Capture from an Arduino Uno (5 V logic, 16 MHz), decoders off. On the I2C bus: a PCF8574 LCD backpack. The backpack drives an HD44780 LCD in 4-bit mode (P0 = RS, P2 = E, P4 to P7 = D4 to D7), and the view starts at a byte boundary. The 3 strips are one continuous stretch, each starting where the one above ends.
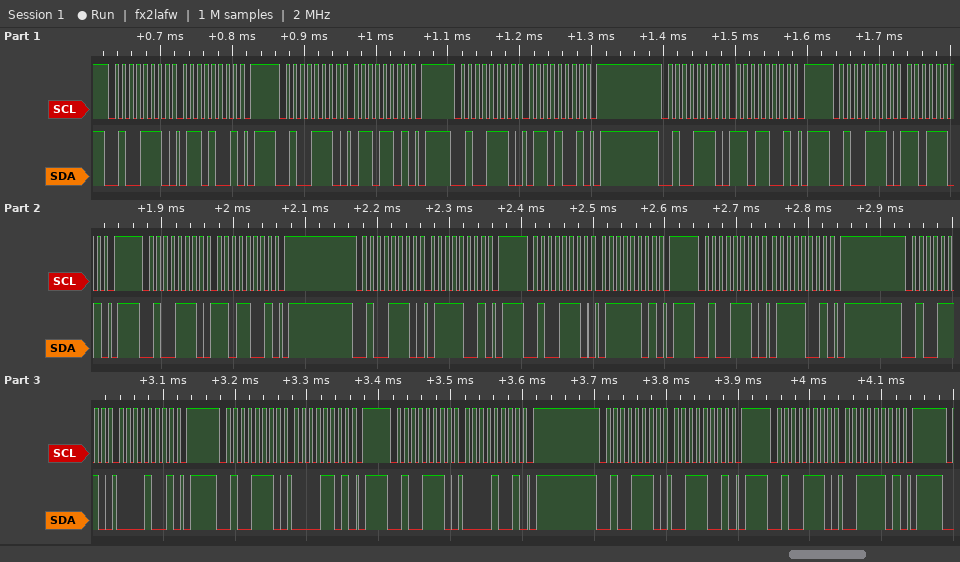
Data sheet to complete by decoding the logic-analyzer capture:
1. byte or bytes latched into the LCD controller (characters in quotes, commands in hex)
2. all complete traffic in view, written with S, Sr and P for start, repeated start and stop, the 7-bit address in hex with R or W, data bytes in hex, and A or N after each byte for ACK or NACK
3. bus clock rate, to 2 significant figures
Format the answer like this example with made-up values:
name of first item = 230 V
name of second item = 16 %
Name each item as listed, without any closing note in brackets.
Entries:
byte or bytes latched into the LCD controller = 'm' 'p'
all complete traffic in view, written with S, Sr and P for start, repeated start and stop, the 7-bit address in hex with R or W, data bytes in hex, and A or N after each byte for ACK or NACK = S 27W A 69 A P S 27W A 6D A P S 27W A 69 A P S 27W A D9 A P S 27W A DD A P S 27W A D9 A P S 27W A 79 A P S 27W A 7D A P S 27W A 79 A P S 27W A 09 A P S 27W A 0D A P S 27W A 09 A P S 27W A 39 A P S 27W A 3D A P
bus clock rate, to 2 significant figures = 100 kHz
